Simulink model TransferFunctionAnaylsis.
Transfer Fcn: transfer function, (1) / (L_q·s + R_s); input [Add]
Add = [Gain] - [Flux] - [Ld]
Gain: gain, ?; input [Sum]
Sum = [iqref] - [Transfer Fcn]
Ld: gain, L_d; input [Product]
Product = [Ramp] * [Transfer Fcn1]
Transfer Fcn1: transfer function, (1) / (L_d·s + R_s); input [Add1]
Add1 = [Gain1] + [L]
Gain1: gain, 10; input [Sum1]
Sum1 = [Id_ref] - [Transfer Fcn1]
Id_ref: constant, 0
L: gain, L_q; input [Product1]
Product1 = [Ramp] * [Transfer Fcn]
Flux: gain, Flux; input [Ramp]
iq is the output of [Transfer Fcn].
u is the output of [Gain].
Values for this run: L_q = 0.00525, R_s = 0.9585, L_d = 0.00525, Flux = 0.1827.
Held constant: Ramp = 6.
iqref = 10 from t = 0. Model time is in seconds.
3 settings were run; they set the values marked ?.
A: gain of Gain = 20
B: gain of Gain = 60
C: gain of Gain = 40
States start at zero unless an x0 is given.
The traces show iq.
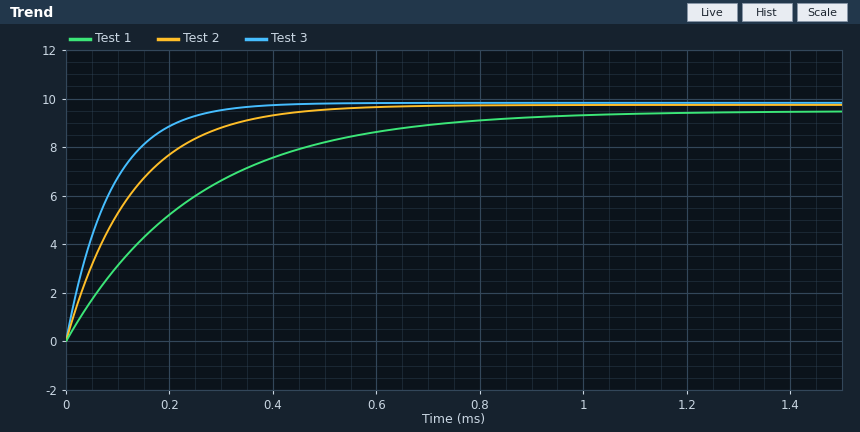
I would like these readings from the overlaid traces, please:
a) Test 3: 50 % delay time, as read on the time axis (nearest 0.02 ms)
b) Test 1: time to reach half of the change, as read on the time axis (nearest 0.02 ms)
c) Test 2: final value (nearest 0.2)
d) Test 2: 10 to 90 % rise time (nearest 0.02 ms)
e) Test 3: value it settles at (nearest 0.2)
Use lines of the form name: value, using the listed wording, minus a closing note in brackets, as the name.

Test 3: 50 % delay time, as read on the time axis: 0.06 ms
Test 1: time to reach half of the change, as read on the time axis: 0.18 ms
Test 2: final value: 9.8
Test 2: 10 to 90 % rise time: 0.28 ms
Test 3: value it settles at: 9.8
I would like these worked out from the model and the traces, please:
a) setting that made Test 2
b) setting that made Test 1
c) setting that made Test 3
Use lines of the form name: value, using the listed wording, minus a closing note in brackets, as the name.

setting that made Test 2: C
setting that made Test 1: A
setting that made Test 3: B
